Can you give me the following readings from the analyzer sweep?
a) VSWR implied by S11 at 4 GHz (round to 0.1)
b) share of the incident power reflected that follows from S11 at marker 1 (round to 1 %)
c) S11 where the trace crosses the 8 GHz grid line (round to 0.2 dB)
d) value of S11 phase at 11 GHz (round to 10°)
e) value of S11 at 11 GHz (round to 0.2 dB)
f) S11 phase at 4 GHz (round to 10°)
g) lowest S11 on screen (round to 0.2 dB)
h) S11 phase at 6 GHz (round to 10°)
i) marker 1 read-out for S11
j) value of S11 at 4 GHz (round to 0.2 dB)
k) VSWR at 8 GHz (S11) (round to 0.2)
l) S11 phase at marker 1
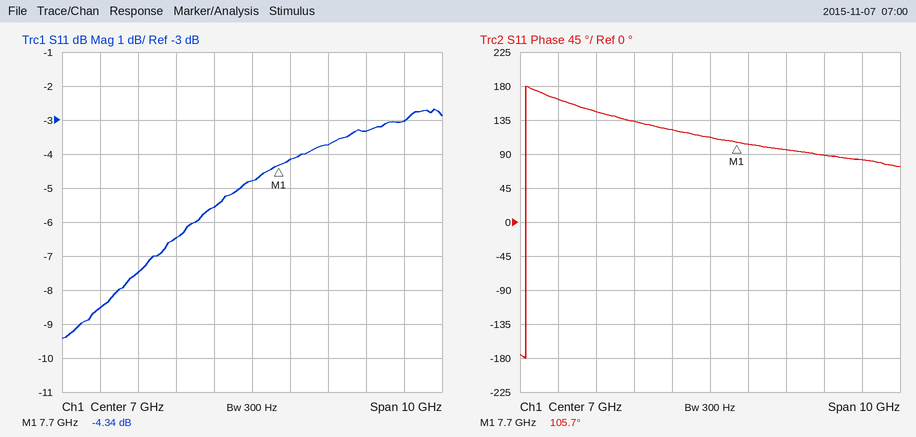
2.5
37 %
-4.2 dB
80°
-3.0 dB
150°
-9.4 dB
120°
-4.34 dB
-7.4 dB
4.2
105.7°
